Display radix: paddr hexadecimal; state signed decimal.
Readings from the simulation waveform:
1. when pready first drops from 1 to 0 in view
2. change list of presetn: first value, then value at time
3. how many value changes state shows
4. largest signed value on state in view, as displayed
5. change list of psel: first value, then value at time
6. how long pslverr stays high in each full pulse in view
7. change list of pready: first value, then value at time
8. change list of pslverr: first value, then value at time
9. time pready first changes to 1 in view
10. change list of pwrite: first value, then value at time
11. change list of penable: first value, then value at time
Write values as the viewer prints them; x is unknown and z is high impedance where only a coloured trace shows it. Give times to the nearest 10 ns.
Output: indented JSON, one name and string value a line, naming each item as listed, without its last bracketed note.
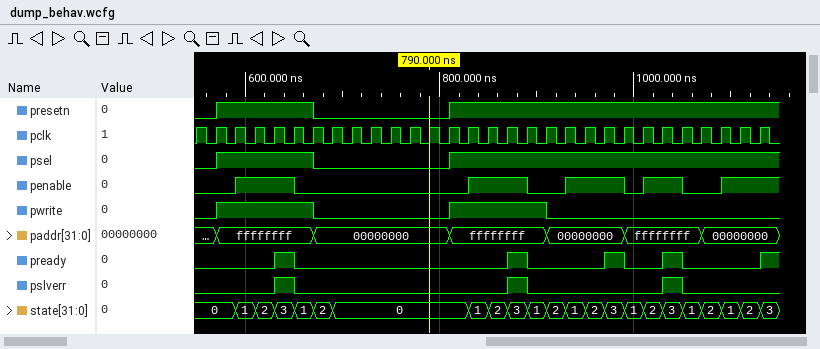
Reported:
{
  "when pready first drops from 1 to 0 in view": "650 ns",
  "change list of presetn: first value, then value at time": "0, 1 at 570 ns, 0 at 670 ns, 1 at 810 ns",
  "how many value changes state shows": "22",
  "largest signed value on state in view, as displayed": "3",
  "change list of psel: first value, then value at time": "0, 1 at 570 ns, 0 at 670 ns, 1 at 810 ns",
  "how long pslverr stays high in each full pulse in view": "20 ns, 20 ns, 20 ns",
  "change list of pready: first value, then value at time": "0, 1 at 630 ns, 0 at 650 ns, 1 at 870 ns, 0 at 890 ns, 1 at 970 ns, 0 at 990 ns, 1 at 1030 ns, 0 at 1050 ns, 1 at 1130 ns",
  "change list of pslverr: first value, then value at time": "0, 1 at 630 ns, 0 at 650 ns, 1 at 870 ns, 0 at 890 ns, 1 at 1030 ns, 0 at 1050 ns",
  "time pready first changes to 1 in view": "630 ns",
  "change list of pwrite: first value, then value at time": "0, 1 at 570 ns, 0 at 670 ns, 1 at 810 ns, 0 at 910 ns",
  "change list of penable: first value, then value at time": "0, 1 at 590 ns, 0 at 650 ns, 1 at 830 ns, 0 at 890 ns, 1 at 930 ns, 0 at 990 ns, 1 at 1010 ns, 0 at 1050 ns, 1 at 1090 ns"
}
